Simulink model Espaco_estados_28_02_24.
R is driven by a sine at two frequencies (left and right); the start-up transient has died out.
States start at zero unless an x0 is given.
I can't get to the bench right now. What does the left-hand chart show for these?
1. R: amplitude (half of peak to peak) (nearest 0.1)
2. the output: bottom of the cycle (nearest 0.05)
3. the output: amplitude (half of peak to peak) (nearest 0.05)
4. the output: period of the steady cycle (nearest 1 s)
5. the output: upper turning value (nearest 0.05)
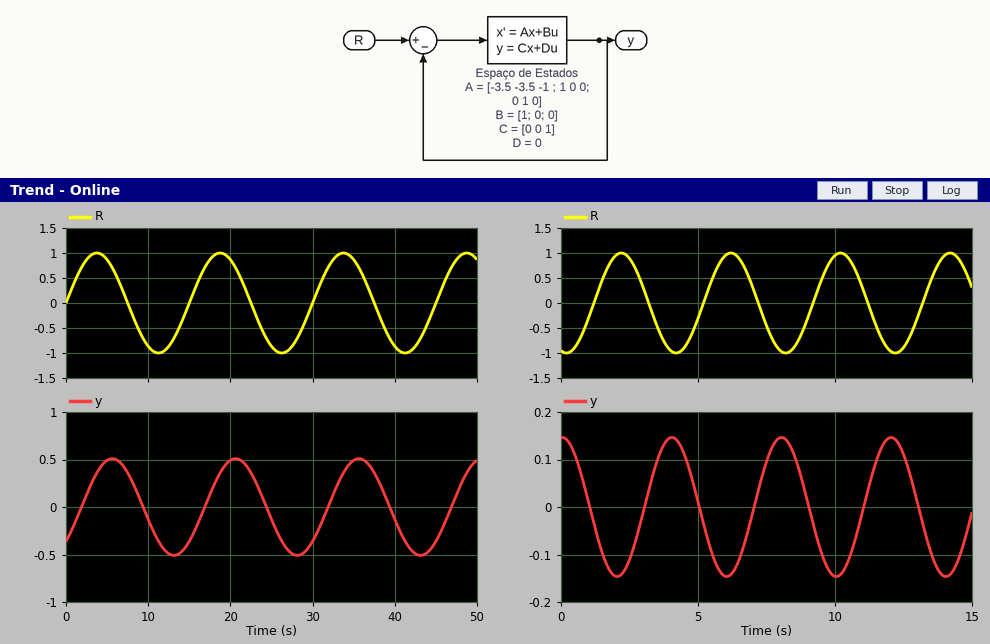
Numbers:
1.0
-0.50
0.50
15 s
0.50
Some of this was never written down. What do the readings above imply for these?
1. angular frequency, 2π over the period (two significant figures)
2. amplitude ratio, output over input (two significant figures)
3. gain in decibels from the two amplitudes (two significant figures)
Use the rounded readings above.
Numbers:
0.42 rad/s
0.50
-6.0 dB
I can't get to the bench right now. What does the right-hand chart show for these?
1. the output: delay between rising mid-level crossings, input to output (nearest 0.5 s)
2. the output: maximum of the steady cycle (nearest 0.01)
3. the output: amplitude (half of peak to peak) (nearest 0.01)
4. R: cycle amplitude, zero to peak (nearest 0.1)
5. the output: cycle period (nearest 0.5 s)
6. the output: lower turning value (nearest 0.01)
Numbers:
2.0 s
0.15
0.15
1.0
4.0 s
-0.15
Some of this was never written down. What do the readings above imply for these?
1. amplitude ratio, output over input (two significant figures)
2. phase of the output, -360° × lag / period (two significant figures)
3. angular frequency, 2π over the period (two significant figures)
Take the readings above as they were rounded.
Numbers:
0.15
-180°
1.6 rad/s
